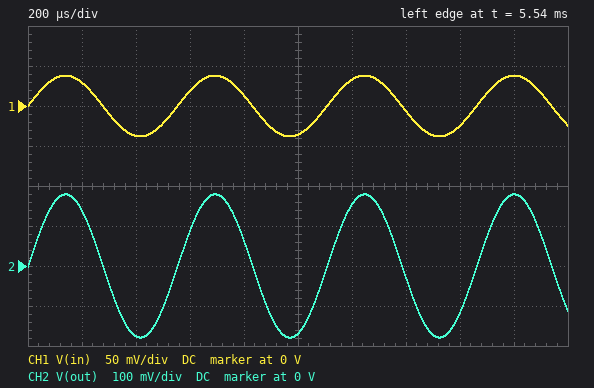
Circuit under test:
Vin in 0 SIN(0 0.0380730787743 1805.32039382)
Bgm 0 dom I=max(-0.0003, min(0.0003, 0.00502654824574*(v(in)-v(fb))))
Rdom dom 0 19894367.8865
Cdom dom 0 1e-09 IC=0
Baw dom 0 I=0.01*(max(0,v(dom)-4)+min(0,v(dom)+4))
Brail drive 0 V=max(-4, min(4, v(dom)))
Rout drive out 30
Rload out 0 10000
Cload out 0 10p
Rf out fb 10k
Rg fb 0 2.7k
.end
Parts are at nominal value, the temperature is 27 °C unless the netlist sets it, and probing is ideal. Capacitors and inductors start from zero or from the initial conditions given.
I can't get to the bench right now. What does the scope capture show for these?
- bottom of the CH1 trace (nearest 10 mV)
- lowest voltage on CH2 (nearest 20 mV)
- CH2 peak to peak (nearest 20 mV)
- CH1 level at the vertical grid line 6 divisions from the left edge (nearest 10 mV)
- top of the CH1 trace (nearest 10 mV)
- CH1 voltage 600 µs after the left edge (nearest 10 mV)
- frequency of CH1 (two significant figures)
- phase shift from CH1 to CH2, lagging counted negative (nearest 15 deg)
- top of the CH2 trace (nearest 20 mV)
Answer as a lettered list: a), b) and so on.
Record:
a) -40 mV
b) -180 mV
c) 360 mV
d) 30 mV
e) 40 mV
f) 20 mV
g) 1.8 kHz
h) 0 deg
i) 180 mV
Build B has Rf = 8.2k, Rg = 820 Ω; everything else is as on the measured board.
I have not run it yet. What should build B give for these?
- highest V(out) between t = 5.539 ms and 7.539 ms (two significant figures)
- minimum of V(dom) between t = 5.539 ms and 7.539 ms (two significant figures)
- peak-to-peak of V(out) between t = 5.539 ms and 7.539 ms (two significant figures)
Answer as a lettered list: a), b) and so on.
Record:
a) 420 mV
b) -420 mV
c) 840 mV
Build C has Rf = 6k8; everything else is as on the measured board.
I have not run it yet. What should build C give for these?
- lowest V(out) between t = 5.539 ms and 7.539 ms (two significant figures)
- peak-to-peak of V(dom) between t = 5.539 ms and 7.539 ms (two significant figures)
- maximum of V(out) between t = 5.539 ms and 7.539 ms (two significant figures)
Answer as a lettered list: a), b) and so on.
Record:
a) -130 mV
b) 270 mV
c) 130 mV
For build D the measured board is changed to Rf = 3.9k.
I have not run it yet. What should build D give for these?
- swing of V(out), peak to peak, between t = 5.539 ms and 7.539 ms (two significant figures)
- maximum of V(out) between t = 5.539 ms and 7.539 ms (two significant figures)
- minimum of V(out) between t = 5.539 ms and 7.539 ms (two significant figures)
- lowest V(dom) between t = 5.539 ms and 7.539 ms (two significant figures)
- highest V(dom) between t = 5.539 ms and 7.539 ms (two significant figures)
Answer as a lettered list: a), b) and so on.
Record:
a) 190 mV
b) 93 mV
c) -93 mV
d) -94 mV
e) 94 mV
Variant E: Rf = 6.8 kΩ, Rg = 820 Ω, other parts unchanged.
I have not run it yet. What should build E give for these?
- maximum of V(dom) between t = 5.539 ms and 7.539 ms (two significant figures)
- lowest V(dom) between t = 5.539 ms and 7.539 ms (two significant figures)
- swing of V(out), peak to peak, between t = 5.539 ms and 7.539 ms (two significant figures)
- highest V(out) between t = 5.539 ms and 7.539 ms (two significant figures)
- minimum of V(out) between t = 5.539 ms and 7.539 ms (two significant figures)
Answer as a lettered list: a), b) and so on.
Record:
a) 360 mV
b) -360 mV
c) 710 mV
d) 350 mV
e) -350 mV
